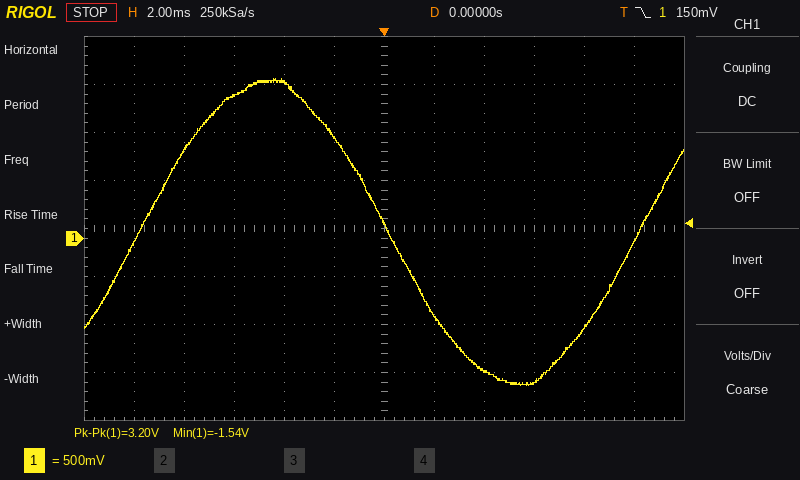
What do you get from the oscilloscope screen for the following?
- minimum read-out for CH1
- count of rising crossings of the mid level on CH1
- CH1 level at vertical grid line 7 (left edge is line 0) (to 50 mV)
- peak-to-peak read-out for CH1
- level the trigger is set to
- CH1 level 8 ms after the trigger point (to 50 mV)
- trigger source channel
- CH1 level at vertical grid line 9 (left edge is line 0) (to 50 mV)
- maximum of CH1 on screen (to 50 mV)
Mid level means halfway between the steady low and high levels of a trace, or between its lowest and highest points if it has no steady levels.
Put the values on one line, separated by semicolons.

-1.54 V; 2; -800 mV; 3.20 V; 150 mV; -950 mV; CH1; -1.50 V; 1.65 V
